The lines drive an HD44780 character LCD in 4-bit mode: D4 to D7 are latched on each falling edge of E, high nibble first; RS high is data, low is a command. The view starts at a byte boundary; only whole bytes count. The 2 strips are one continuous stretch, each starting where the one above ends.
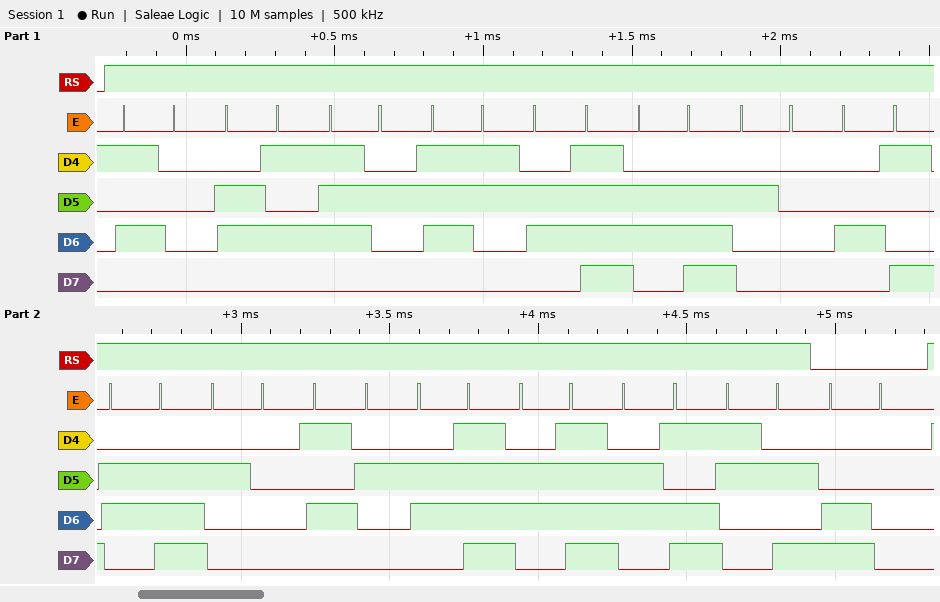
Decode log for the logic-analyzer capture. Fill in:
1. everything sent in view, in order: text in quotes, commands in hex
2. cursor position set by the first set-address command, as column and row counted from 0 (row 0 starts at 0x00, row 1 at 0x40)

"Person In Room:" 0xC0
column 0, row 1
